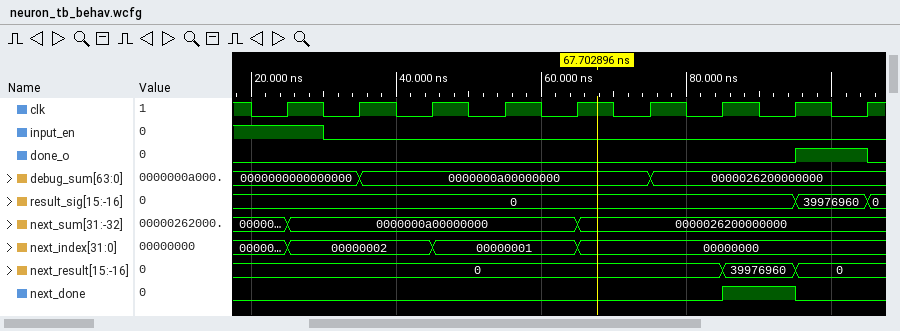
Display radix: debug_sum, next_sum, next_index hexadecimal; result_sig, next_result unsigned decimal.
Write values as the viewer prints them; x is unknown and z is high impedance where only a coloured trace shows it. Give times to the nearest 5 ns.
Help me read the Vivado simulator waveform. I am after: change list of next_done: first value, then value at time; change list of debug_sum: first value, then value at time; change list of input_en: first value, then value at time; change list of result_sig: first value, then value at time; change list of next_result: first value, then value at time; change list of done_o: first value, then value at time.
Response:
0, 1 at 85 ns, 0 at 95 ns
0000000000000000, 0000000a00000000 at 35 ns, 0000026200000000 at 75 ns
1, 0 at 30 ns
0, 39976960 at 95 ns, 0 at 105 ns
0, 39976960 at 85 ns, 0 at 95 ns
0, 1 at 95 ns, 0 at 105 ns
